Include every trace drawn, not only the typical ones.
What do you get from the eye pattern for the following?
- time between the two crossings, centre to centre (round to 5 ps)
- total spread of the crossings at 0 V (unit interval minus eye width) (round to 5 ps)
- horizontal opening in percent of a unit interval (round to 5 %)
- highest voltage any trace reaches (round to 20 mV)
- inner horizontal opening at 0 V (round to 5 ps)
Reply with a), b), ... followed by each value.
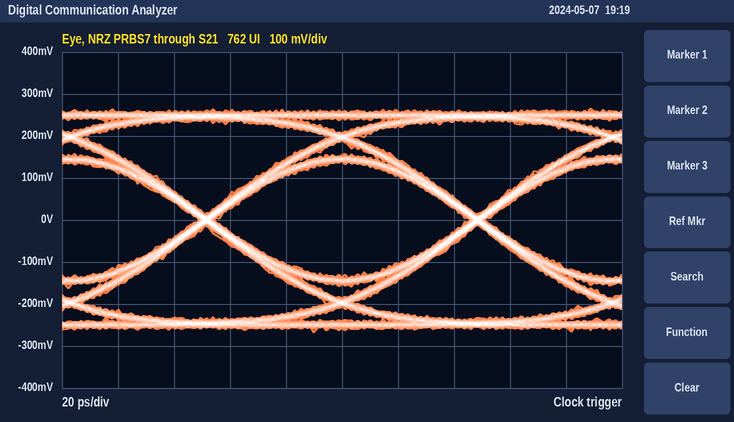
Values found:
a) 95 ps
b) 5 ps
c) 95 %
d) 260 mV
e) 90 ps
